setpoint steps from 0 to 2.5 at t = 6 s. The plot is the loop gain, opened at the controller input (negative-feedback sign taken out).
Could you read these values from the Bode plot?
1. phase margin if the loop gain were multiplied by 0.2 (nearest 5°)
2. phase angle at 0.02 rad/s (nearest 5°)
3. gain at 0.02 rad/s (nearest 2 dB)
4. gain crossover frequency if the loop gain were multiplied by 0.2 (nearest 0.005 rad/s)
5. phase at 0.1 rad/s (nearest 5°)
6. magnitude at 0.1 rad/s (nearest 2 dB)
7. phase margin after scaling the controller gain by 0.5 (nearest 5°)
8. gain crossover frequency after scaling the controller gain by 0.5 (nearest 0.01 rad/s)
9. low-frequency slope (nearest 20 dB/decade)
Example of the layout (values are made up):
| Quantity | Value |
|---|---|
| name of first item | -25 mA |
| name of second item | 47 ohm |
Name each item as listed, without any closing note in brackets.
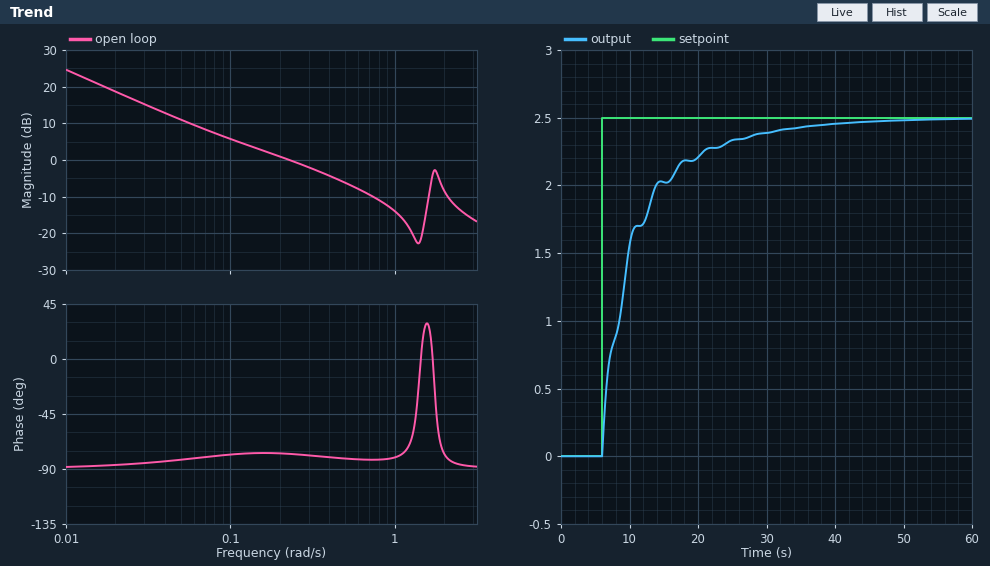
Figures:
| Quantity | Value |
|---|---|
| phase margin if the loop gain were multiplied by 0.2 | 95° |
| phase angle at 0.02 rad/s | -85° |
| gain at 0.02 rad/s | 18 dB |
| gain crossover frequency if the loop gain were multiplied by 0.2 | 0.035 rad/s |
| phase at 0.1 rad/s | -80° |
| magnitude at 0.1 rad/s | 6 dB |
| phase margin after scaling the controller gain by 0.5 | 100° |
| gain crossover frequency after scaling the controller gain by 0.5 | 0.10 rad/s |
| low-frequency slope | -20 dB/decade |
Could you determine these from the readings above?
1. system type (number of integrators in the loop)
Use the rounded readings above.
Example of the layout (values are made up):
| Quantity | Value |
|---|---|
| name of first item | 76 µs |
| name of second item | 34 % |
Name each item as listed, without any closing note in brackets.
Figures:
| Quantity | Value |
|---|---|
| system type | 1 |
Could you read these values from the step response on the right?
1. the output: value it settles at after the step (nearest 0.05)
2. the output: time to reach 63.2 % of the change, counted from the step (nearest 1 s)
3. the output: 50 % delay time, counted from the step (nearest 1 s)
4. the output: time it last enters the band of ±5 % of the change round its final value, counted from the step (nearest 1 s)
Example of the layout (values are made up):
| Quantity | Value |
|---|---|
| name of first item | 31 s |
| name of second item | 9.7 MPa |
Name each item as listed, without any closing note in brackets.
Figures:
| Quantity | Value |
|---|---|
| the output: value it settles at after the step | 2.50 |
| the output: time to reach 63.2 % of the change, counted from the step | 4 s |
| the output: 50 % delay time, counted from the step | 3 s |
| the output: time it last enters the band of ±5 % of the change round its final value, counted from the step | 22 s |
